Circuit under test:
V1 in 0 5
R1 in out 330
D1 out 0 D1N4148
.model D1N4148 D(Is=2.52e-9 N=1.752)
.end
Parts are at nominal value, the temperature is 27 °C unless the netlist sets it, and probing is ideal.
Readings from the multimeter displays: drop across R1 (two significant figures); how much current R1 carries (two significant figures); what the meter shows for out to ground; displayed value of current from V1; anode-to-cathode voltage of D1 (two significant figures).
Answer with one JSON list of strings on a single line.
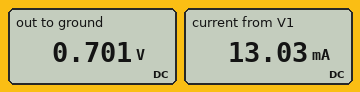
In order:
["4.3 V", "13 mA", "0.701 V", "13.03 mA", "700 mV"]
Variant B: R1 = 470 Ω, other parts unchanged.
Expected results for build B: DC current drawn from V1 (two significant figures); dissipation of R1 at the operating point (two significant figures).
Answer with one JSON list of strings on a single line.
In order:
["9.2 mA", "40 mW"]
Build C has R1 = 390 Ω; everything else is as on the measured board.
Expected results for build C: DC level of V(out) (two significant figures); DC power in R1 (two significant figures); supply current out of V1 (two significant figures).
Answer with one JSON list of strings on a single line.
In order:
["690 mV", "48 mW", "11 mA"]
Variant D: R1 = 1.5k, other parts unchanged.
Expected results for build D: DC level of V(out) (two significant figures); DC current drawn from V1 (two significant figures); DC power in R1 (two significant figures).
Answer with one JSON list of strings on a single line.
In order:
["630 mV", "2.9 mA", "13 mW"]
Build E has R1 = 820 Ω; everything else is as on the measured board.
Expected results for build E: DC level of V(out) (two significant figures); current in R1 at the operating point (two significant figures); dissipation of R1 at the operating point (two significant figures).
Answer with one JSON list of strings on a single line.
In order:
["660 mV", "5.3 mA", "23 mW"]
